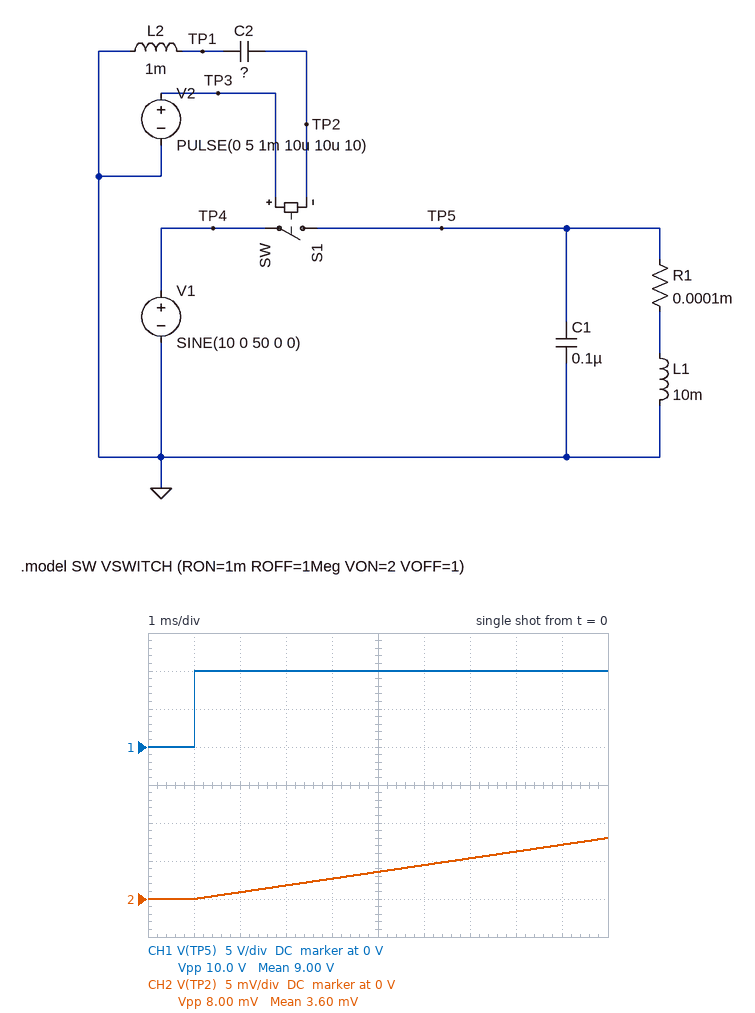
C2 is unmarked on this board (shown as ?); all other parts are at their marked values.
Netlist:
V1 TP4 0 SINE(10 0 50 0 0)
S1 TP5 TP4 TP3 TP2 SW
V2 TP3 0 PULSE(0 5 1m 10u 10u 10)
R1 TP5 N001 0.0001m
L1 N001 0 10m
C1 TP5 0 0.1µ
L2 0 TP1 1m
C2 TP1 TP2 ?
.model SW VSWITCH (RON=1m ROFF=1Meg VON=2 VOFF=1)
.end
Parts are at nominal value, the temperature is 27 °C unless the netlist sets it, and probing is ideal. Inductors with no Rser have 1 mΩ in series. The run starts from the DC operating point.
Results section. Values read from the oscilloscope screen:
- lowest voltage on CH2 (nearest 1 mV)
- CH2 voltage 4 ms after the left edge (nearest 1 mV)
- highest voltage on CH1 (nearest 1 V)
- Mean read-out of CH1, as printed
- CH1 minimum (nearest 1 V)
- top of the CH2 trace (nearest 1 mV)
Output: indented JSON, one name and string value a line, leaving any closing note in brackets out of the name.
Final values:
{
  "lowest voltage on CH2": "0 V",
  "CH2 voltage 4 ms after the left edge": "3 mV",
  "highest voltage on CH1": "10 V",
  "Mean read-out of CH1, as printed": "9.00 V",
  "CH1 minimum": "0 V",
  "top of the CH2 trace": "8 mV"
}
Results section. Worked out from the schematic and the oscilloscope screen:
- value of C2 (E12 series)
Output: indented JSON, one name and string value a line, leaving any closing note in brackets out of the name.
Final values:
{
  "value of C2": "5.6 pF"
}
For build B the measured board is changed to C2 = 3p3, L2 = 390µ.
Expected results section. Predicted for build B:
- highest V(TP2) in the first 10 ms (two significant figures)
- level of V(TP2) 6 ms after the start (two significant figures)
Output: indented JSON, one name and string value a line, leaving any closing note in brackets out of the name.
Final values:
{
  "highest V(TP2) in the first 10 ms": "14 mV",
  "level of V(TP2) 6 ms after the start": "7.6 mV"
}
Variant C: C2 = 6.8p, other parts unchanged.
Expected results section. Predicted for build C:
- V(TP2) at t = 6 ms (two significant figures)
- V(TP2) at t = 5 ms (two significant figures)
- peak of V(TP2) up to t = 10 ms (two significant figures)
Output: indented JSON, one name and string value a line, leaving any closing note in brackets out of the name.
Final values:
{
  "V(TP2) at t = 6 ms": "3.7 mV",
  "V(TP2) at t = 5 ms": "2.9 mV",
  "peak of V(TP2) up to t = 10 ms": "6.6 mV"
}
